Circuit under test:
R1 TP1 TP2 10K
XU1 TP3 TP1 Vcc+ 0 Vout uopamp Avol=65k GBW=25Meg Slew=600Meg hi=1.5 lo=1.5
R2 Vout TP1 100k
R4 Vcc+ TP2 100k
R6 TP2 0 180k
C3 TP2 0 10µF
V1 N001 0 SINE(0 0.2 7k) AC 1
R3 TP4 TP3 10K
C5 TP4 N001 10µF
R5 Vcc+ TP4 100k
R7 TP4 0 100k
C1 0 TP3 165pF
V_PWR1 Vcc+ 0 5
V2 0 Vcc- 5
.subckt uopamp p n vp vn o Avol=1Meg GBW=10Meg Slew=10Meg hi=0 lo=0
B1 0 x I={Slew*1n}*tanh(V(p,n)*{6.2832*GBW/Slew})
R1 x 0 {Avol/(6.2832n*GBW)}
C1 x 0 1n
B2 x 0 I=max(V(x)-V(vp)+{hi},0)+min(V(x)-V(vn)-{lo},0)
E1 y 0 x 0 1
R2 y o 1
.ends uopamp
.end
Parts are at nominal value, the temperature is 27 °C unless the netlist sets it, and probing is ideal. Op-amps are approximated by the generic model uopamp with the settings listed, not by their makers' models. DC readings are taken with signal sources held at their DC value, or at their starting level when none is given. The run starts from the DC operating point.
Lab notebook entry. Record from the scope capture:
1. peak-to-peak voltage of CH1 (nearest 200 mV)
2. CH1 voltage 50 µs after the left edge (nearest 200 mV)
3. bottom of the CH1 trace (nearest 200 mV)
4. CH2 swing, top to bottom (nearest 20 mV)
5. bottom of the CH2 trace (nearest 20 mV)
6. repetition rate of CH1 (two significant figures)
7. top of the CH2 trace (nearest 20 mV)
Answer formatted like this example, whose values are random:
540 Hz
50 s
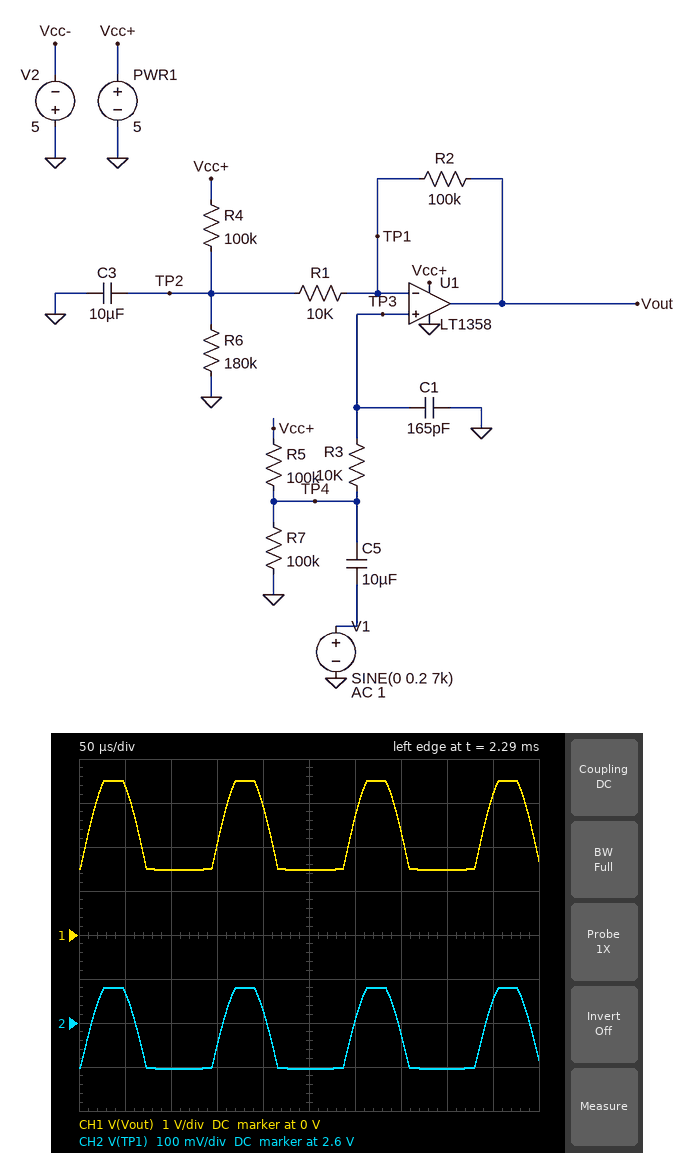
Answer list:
2.0 V
3.4 V
1.4 V
180 mV
2.50 V
7.0 kHz
2.68 V
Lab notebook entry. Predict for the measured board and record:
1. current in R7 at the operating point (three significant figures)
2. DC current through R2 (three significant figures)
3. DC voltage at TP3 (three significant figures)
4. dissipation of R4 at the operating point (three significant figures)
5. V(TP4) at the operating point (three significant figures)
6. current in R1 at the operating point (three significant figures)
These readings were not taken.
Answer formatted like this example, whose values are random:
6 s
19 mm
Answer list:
25.0 µA
9.62 µA
2.50 V
57.8 µW
2.50 V
9.62 µA
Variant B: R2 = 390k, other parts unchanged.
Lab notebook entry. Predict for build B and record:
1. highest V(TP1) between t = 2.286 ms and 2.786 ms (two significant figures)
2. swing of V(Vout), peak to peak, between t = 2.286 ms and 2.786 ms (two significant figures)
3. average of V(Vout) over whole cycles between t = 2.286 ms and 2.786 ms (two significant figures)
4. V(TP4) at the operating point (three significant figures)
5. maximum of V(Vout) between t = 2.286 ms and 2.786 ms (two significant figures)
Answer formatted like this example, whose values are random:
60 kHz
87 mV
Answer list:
2.9 V
62 mV
1.4 V
2.50 V
1.5 V
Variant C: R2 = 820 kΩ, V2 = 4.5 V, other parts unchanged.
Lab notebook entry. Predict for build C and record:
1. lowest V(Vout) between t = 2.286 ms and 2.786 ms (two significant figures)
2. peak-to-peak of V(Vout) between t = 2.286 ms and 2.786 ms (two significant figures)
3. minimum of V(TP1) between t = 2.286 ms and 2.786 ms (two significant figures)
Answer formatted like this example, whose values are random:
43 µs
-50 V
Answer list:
1.4 V
61 mV
3.1 V
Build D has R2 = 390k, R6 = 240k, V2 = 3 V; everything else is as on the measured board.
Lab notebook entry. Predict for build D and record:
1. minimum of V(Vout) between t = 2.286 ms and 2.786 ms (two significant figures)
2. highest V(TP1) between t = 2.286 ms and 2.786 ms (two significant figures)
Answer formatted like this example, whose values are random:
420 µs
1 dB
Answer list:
1.4 V
3.2 V
